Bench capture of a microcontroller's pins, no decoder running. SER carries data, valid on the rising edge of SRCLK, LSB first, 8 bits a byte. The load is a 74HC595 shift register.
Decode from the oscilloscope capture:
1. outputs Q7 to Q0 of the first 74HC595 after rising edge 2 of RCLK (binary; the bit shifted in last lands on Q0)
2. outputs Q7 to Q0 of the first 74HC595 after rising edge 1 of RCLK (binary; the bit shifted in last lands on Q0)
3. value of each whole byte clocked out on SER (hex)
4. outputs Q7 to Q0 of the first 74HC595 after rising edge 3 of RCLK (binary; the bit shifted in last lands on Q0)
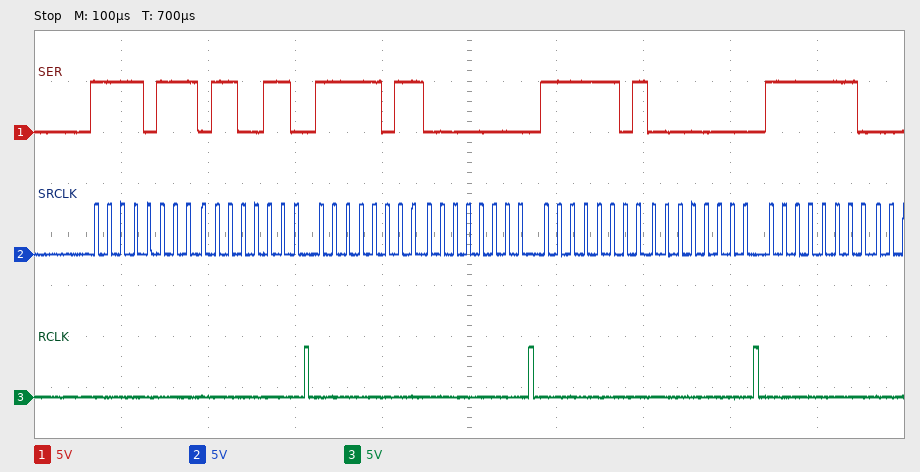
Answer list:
00000000
01100110
EF 66 DF 00 BF 00 7F
00000000
